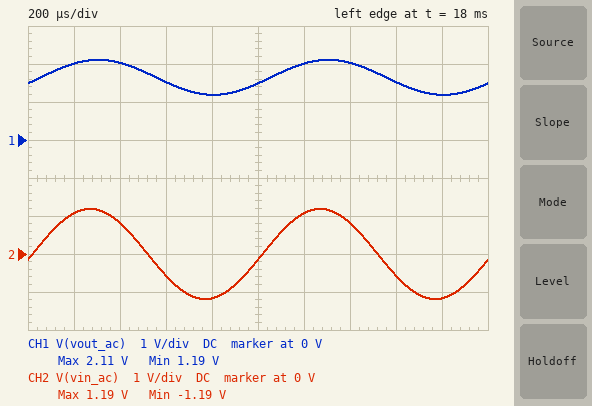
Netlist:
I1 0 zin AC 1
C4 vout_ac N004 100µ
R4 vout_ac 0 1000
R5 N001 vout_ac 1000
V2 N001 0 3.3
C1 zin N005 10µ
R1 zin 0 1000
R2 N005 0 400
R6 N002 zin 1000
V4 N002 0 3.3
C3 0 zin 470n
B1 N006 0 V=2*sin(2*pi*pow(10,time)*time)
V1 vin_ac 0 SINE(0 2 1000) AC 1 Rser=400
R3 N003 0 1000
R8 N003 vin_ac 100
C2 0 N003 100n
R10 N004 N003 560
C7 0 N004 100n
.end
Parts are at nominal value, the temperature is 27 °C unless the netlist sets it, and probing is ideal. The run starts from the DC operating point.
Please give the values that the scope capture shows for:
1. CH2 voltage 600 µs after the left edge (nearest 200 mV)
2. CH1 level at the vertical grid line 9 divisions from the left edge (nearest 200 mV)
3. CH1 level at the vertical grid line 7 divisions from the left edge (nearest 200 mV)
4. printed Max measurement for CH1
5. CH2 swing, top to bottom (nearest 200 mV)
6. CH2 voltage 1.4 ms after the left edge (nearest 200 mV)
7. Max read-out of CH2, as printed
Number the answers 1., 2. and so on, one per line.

1. -600 mV
2. 1.2 V
3. 2.0 V
4. 2.11 V
5. 2.4 V
6. 800 mV
7. 1.19 V
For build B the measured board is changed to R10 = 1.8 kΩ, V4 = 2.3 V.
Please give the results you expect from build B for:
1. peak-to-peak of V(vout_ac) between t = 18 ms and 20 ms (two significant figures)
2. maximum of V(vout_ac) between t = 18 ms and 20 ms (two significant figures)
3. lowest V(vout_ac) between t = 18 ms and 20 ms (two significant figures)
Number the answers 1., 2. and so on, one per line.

1. 480 mV
2. 1.9 V
3. 1.4 V
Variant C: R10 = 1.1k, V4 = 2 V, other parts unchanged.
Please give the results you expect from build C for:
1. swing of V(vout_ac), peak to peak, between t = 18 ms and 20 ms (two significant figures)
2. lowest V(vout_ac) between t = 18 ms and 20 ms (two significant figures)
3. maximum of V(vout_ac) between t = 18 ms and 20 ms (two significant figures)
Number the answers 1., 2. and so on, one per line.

1. 660 mV
2. 1.3 V
3. 2.0 V
